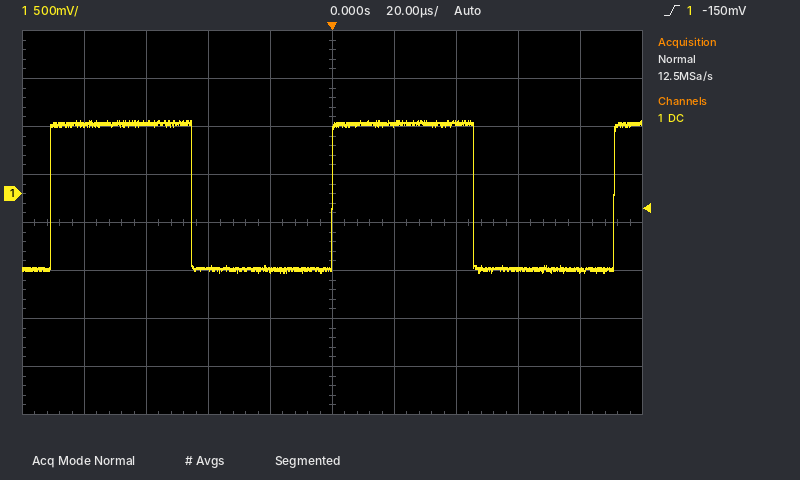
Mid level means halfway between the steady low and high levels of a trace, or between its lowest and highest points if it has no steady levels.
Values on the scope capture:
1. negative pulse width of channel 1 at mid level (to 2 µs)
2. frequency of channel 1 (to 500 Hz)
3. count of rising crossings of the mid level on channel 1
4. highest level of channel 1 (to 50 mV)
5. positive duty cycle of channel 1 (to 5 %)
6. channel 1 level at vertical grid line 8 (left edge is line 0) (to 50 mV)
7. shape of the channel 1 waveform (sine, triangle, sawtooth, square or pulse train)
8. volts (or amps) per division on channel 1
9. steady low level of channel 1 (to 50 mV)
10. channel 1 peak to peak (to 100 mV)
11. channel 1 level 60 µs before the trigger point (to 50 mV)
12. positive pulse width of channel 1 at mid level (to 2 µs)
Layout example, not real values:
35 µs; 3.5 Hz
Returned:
46 µs; 11.0 kHz; 3; 750 mV; 50 %; -800 mV; square; 500 mV; -800 mV; 1.60 V; 750 mV; 46 µs
